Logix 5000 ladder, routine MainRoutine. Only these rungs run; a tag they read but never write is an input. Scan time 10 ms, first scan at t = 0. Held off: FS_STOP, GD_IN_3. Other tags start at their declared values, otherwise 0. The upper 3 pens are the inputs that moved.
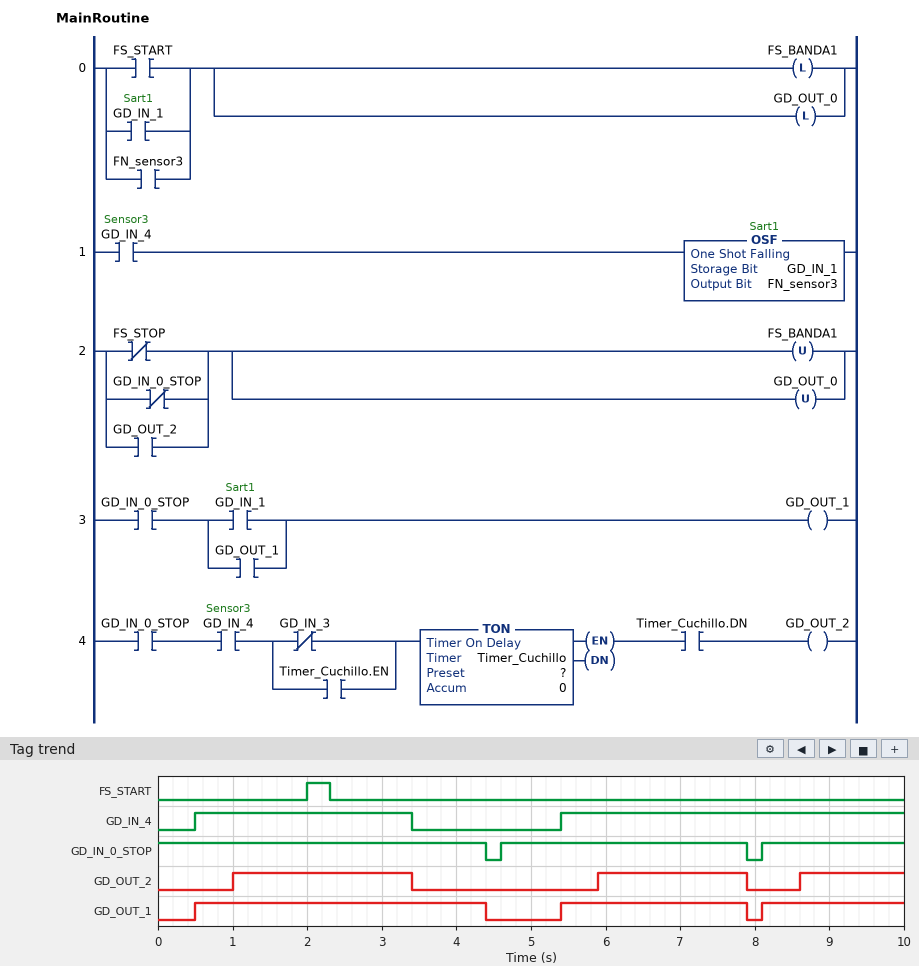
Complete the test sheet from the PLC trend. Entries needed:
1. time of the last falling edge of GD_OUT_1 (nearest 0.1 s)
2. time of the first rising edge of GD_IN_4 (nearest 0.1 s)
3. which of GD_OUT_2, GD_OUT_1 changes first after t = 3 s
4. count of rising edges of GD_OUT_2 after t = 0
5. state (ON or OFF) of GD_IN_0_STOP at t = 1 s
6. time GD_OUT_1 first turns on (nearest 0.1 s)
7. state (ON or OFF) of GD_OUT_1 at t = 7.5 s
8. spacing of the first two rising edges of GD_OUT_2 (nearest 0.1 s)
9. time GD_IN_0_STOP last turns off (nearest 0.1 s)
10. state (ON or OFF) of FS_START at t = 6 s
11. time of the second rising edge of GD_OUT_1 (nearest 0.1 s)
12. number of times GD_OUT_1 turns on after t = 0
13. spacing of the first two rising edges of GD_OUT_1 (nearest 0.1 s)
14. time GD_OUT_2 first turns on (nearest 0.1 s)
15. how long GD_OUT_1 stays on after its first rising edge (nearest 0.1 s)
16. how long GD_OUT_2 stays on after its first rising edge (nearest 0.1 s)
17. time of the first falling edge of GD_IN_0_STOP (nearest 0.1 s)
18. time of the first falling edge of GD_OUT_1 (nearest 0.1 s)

7.9 s
0.5 s
GD_OUT_2
3
ON
0.5 s
ON
4.9 s
7.9 s
OFF
5.4 s
3
4.9 s
1.0 s
3.9 s
2.4 s
4.4 s
4.4 s
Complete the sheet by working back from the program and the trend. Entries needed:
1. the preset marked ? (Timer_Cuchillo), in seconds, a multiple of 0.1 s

0.5 s
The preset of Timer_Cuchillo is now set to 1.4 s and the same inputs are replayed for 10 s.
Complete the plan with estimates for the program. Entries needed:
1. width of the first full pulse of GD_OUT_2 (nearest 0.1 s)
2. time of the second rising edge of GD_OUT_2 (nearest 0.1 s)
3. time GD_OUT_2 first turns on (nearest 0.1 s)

1.5 s
6.8 s
1.9 s
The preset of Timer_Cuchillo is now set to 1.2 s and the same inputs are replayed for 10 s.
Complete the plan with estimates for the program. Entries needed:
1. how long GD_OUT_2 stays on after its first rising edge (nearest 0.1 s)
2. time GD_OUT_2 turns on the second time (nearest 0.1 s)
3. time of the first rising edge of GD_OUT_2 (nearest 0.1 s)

1.7 s
6.6 s
1.7 s
